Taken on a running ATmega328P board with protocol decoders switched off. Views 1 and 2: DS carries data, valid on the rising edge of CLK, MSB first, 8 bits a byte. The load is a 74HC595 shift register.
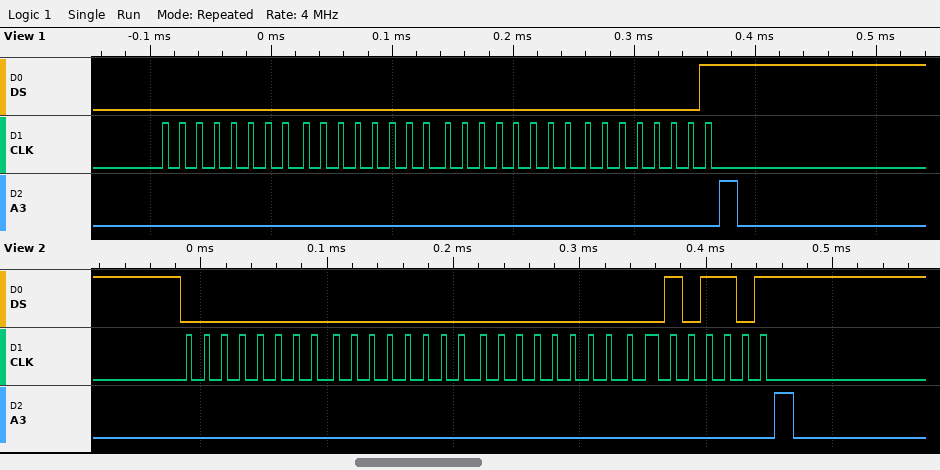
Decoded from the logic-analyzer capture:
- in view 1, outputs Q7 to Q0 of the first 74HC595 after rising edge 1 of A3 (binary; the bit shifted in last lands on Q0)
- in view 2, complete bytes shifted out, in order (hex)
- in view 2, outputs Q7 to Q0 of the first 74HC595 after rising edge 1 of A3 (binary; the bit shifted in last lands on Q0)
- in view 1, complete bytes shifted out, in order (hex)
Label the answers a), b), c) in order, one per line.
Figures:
a) 00000001
b) 00 00 00 2D
c) 00101101
d) 00 00 00 01
